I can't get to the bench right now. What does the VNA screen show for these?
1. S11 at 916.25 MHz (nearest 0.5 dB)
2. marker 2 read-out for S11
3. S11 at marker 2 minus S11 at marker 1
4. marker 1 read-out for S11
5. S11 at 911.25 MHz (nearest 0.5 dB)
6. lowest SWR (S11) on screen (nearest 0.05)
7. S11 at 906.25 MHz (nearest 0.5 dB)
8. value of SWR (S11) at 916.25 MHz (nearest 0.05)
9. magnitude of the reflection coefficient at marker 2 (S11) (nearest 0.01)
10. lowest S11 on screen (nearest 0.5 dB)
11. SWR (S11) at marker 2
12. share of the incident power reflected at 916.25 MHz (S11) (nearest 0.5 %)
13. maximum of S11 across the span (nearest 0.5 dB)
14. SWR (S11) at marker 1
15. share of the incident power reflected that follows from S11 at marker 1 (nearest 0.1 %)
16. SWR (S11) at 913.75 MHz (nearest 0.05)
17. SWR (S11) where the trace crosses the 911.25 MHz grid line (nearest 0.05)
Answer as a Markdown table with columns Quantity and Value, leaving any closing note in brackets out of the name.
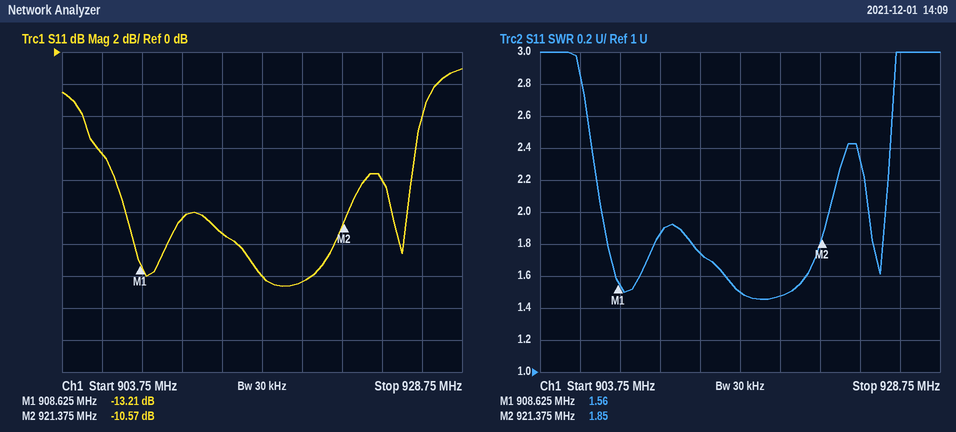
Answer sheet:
| Quantity | Value |
|---|---|
| S11 at 916.25 MHz | -14.0 dB |
| marker 2 read-out for S11 | -10.57 dB |
| S11 at marker 2 minus S11 at marker 1 | 2.64 dB |
| marker 1 read-out for S11 | -13.21 dB |
| S11 at 911.25 MHz | -10.5 dB |
| lowest SWR (S11) on screen | 1.45 |
| S11 at 906.25 MHz | -6.5 dB |
| value of SWR (S11) at 916.25 MHz | 1.50 |
| magnitude of the reflection coefficient at marker 2 (S11) | 0.30 |
| lowest S11 on screen | -14.5 dB |
| SWR (S11) at marker 2 | 1.85 |
| share of the incident power reflected at 916.25 MHz (S11) | 4.0 % |
| maximum of S11 across the span | -1.0 dB |
| SWR (S11) at marker 1 | 1.56 |
| share of the incident power reflected that follows from S11 at marker 1 | 4.8 % |
| SWR (S11) at 913.75 MHz | 1.75 |
| SWR (S11) where the trace crosses the 911.25 MHz grid line | 1.85 |
